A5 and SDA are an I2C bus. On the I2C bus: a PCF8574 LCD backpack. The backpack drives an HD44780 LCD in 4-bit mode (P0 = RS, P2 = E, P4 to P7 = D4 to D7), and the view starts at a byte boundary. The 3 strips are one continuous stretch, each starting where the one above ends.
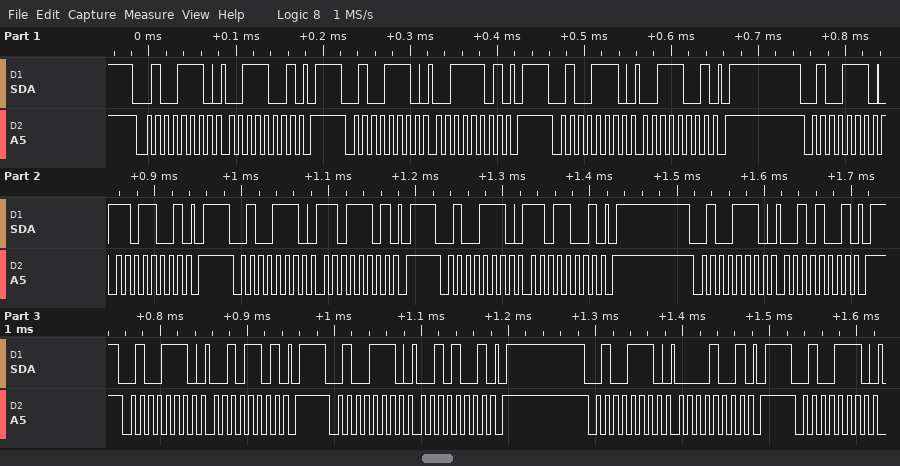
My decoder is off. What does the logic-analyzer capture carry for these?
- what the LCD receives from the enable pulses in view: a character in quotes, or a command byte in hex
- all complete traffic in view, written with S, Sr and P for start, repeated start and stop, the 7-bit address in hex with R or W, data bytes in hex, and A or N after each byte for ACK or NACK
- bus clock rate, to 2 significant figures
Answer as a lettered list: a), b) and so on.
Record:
a) '='
b) S 27W A 39 A P S 27W A 3D A P S 27W A 39 A P S 27W A D9 A P S 27W A DD A P S 27W A D9 A P S 27W A 29 A P S 27W A 2D A P S 27W A 29 A P S 27W A 09 A P S 27W A
c) 100 kHz
